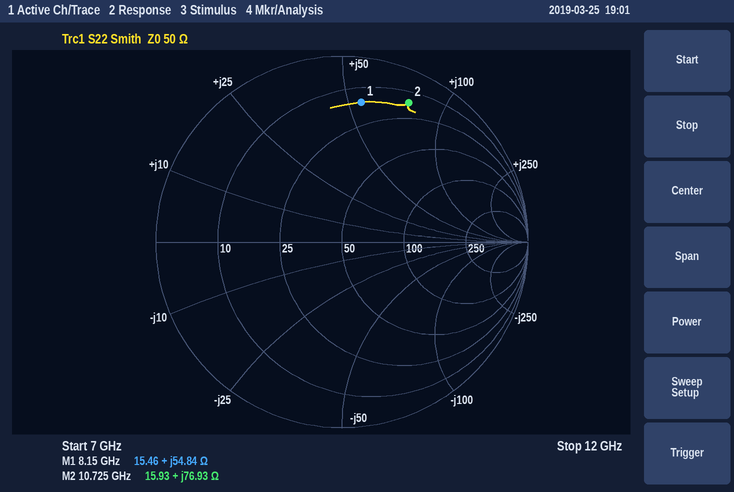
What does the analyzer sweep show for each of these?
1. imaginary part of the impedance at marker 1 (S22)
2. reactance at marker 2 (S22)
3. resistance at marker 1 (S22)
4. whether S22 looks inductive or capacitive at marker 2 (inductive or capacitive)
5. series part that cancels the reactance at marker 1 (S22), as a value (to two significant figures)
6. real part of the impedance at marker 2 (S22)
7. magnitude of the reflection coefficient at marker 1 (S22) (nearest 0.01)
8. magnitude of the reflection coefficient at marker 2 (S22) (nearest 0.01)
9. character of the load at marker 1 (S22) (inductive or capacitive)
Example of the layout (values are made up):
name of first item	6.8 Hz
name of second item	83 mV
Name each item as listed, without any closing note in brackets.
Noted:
imaginary part of the impedance at marker 1	+54.84 Ω
reactance at marker 2	+76.93 Ω
resistance at marker 1	15.46 Ω
whether S22 looks inductive or capacitive at marker 2	inductive
series part that cancels the reactance at marker 1 (S22), as a value	360 fF
real part of the impedance at marker 2	15.93 Ω
magnitude of the reflection coefficient at marker 1 (S22)	0.76
magnitude of the reflection coefficient at marker 2 (S22)	0.83
character of the load at marker 1 (S22)	inductive
